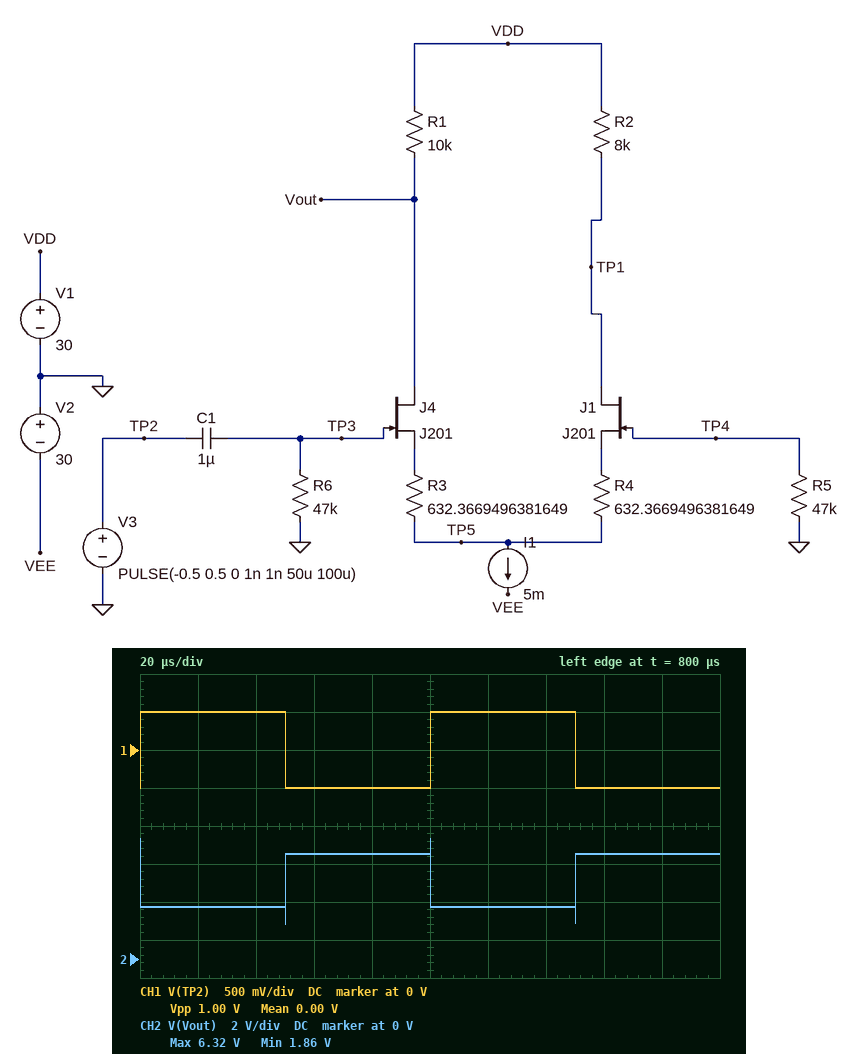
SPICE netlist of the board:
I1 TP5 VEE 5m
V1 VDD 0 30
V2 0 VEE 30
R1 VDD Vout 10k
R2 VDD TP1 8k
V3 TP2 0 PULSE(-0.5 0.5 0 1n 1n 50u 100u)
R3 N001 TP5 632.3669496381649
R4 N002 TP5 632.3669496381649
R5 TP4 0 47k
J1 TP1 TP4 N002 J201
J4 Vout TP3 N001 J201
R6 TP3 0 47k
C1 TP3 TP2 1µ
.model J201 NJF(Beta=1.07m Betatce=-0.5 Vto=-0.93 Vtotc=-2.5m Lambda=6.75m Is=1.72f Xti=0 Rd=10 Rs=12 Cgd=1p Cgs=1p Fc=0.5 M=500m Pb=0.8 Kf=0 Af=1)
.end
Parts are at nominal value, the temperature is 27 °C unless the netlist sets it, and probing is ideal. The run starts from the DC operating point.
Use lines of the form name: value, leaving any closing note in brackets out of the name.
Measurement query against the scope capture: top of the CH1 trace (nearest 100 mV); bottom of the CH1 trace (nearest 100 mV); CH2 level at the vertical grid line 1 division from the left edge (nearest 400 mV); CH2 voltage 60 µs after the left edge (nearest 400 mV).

top of the CH1 trace: 500 mV
bottom of the CH1 trace: -500 mV
CH2 level at the vertical grid line 1 division from the left edge: 2.8 V
CH2 voltage 60 µs after the left edge: 5.6 V
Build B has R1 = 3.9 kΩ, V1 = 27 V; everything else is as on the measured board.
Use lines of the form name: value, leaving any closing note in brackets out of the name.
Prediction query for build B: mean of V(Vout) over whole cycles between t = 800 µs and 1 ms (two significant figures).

mean of V(Vout) over whole cycles between t = 800 µs and 1 ms: 16 V
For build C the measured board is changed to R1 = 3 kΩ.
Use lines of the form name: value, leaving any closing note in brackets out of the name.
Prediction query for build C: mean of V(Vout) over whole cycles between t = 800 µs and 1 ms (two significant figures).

mean of V(Vout) over whole cycles between t = 800 µs and 1 ms: 22 V
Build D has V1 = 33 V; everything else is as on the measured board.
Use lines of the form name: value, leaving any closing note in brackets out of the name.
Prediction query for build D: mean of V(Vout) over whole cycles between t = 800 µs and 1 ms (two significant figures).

mean of V(Vout) over whole cycles between t = 800 µs and 1 ms: 6.9 V
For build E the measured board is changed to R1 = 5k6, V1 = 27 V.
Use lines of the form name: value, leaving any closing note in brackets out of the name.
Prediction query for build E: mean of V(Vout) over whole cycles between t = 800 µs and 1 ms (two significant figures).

mean of V(Vout) over whole cycles between t = 800 µs and 1 ms: 12 V
